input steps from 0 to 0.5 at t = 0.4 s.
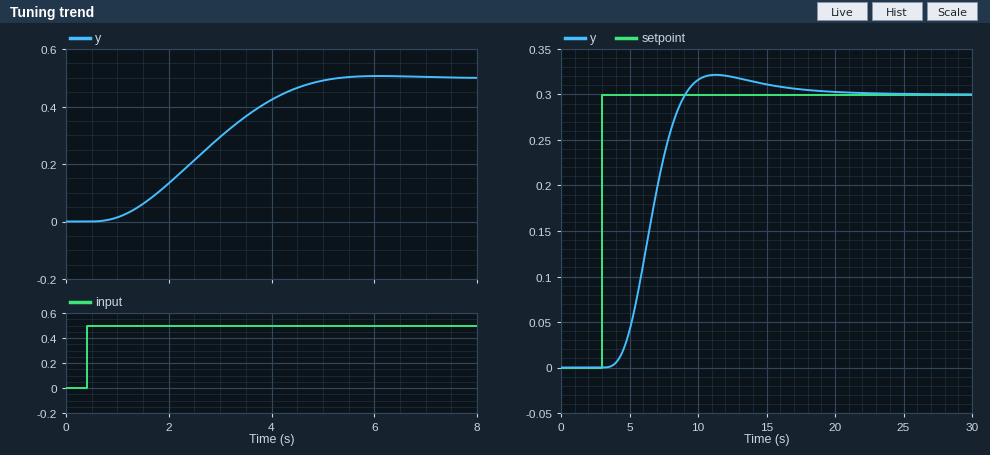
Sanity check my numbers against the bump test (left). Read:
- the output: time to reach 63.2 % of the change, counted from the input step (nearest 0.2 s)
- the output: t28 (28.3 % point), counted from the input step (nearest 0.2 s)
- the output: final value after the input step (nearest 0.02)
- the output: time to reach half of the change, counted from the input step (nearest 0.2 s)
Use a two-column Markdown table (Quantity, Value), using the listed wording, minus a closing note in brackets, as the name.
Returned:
| Quantity | Value |
|---|---|
| the output: time to reach 63.2 % of the change, counted from the input step | 2.8 s |
| the output: t28 (28.3 % point), counted from the input step | 1.6 s |
| the output: final value after the input step | 0.50 |
| the output: time to reach half of the change, counted from the input step | 2.4 s |
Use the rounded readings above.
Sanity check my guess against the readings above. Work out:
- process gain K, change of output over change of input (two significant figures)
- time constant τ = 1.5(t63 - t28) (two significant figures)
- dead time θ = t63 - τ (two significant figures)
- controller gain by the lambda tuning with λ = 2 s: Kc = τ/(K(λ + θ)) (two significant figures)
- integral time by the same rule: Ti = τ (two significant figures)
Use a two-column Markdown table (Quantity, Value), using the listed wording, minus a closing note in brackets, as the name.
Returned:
| Quantity | Value |
|---|---|
| process gain K, change of output over change of input | 1.0 |
| time constant τ = 1.5(t63 - t28) | 1.8 s |
| dead time θ = t63 - τ | 1.0 s |
| controller gain by the lambda tuning with λ = 2 s: Kc = τ/(K(λ + θ)) | 0.60 |
| integral time by the same rule: Ti = τ | 1.8 s |
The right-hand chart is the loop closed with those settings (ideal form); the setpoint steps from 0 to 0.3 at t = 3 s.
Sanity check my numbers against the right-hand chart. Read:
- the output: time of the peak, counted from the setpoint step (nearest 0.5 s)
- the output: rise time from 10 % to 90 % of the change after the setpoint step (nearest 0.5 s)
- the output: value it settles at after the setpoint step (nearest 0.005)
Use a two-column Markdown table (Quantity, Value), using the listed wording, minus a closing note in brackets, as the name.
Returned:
| Quantity | Value |
|---|---|
| the output: time of the peak, counted from the setpoint step | 8.5 s |
| the output: rise time from 10 % to 90 % of the change after the setpoint step | 3.5 s |
| the output: value it settles at after the setpoint step | 0.300 |
